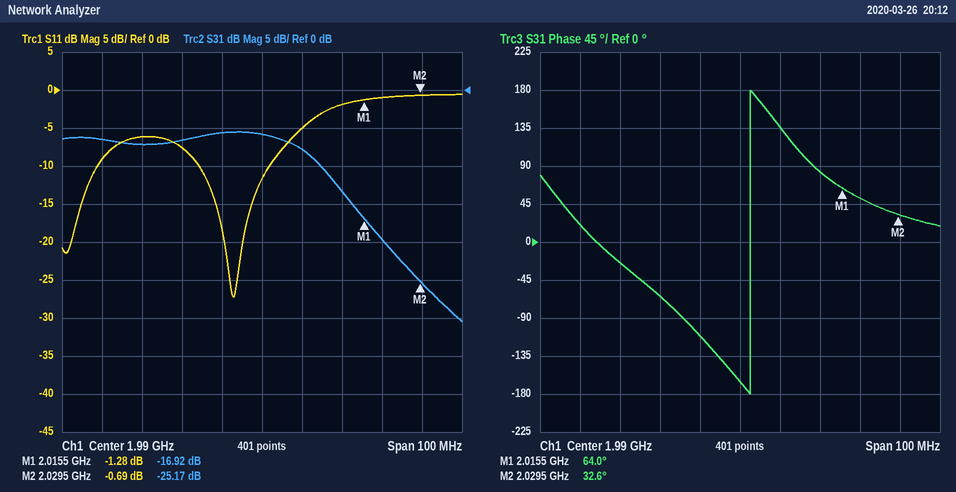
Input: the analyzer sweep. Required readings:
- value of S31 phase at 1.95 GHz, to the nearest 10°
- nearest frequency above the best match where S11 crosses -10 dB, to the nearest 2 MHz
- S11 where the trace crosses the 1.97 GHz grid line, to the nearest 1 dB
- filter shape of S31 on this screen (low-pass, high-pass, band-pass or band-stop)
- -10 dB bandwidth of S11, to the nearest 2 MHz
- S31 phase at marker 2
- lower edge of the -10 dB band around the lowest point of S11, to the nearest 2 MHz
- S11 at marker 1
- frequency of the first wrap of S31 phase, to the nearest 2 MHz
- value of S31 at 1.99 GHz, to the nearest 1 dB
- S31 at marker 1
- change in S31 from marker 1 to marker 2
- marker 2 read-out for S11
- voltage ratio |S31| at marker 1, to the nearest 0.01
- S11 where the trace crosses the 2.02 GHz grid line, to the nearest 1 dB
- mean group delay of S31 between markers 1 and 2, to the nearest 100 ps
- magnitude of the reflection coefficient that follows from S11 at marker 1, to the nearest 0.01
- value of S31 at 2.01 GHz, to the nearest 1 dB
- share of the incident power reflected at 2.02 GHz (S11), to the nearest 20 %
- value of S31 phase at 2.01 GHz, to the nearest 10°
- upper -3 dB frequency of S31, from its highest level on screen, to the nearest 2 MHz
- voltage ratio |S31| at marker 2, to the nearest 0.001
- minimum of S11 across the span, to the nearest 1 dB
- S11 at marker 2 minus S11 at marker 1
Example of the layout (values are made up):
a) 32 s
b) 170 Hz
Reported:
a) 20°
b) 1.992 GHz
c) -8 dB
d) low-pass
e) 18 MHz
f) 32.6°
g) 1.974 GHz
h) -1.28 dB
i) 1.992 GHz
j) -6 dB
k) -16.92 dB
l) -8.25 dB
m) -0.69 dB
n) 0.14
o) -1 dB
p) 6.2 ns
q) 0.86
r) -13 dB
s) 80 %
t) 80°
u) 2.002 GHz
v) 0.055
w) -27 dB
x) 0.59 dB
